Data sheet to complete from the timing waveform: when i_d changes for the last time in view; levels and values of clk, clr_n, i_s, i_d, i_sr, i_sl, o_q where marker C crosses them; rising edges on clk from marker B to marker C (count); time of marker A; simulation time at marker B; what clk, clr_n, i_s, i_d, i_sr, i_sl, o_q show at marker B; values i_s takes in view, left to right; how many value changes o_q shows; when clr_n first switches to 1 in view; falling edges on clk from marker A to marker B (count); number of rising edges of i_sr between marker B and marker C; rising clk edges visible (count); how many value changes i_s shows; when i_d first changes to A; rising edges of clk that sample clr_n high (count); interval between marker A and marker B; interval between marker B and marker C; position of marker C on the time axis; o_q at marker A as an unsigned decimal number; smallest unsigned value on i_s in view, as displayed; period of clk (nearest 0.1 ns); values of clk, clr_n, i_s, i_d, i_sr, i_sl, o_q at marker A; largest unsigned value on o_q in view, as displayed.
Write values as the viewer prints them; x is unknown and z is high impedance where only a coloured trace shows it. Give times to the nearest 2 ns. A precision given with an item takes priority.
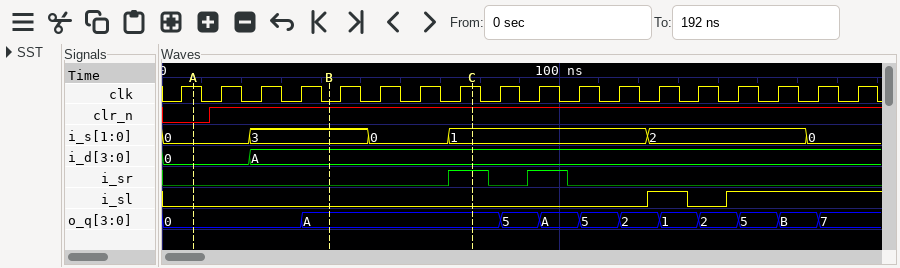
22 ns
clk=1, clr_n=1, i_s=1, i_d=A, i_sr=1, i_sl=0, o_q=A
4
8 ns
42 ns
clk=0, clr_n=1, i_s=3, i_d=A, i_sr=0, i_sl=0, o_q=A
0, 3, 0, 1, 2, 0
10
12 ns
4
1
18
5
22 ns
17
34 ns
36 ns
78 ns
0
0
10 ns
clk=1, clr_n=0, i_s=0, i_d=0, i_sr=0, i_sl=0, o_q=0
B
